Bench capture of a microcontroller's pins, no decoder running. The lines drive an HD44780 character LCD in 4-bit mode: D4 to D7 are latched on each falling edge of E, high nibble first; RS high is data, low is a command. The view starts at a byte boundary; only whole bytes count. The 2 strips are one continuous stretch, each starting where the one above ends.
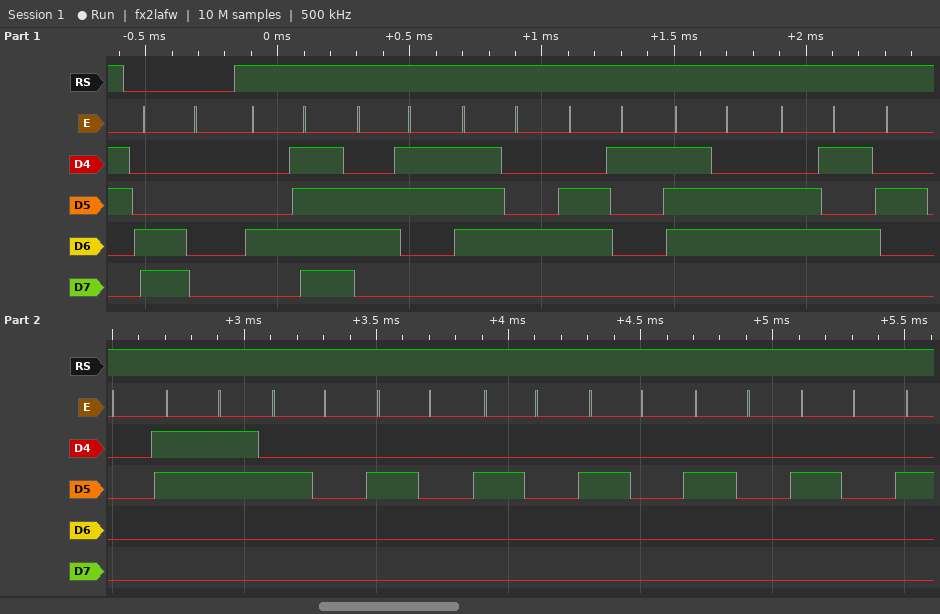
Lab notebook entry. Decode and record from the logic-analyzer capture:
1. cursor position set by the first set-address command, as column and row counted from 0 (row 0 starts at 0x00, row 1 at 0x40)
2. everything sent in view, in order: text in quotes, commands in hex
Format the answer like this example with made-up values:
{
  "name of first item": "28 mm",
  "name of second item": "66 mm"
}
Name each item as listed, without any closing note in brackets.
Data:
{
  "cursor position set by the first set-address command, as column and row counted from 0": "column 0, row 1",
  "everything sent in view, in order: text in quotes, commands in hex": "0xC0 \"Octave 3      \""
}
